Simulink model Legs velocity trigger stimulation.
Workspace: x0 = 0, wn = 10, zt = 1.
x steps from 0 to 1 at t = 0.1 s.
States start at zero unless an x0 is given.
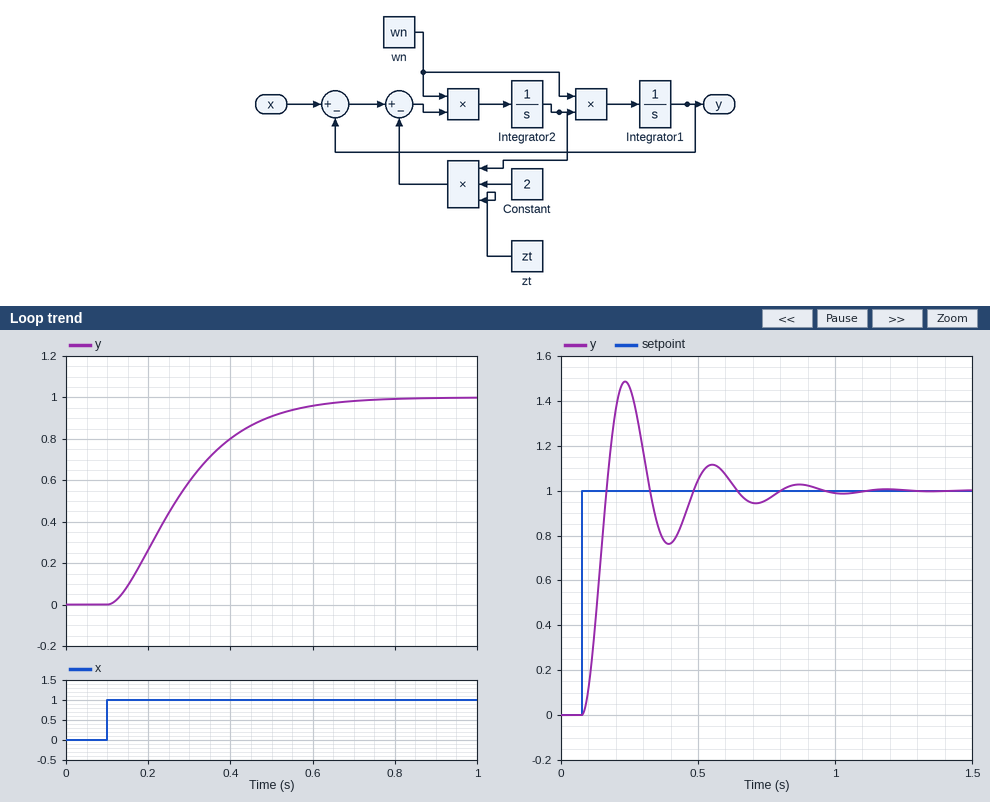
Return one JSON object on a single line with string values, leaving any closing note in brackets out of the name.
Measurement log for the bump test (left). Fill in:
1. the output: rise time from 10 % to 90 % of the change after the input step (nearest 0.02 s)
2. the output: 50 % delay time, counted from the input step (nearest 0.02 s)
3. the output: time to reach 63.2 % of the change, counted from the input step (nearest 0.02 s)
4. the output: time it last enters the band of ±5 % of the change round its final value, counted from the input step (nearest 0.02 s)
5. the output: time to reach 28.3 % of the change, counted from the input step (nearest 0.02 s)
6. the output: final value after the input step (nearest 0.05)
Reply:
{"the output: rise time from 10 % to 90 % of the change after the input step": "0.34 s", "the output: 50 % delay time, counted from the input step": "0.16 s", "the output: time to reach 63.2 % of the change, counted from the input step": "0.22 s", "the output: time it last enters the band of ±5 % of the change round its final value, counted from the input step": "0.48 s", "the output: time to reach 28.3 % of the change, counted from the input step": "0.10 s", "the output: final value after the input step": "1.00"}
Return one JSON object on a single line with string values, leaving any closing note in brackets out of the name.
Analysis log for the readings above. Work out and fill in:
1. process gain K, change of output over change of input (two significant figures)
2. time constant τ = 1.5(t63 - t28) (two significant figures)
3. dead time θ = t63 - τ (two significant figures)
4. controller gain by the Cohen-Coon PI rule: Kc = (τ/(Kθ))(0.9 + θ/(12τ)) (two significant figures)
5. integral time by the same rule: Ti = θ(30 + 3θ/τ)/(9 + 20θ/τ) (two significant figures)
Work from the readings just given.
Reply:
{"process gain K, change of output over change of input": "1.0", "time constant τ = 1.5(t63 - t28)": "0.18 s", "dead time θ = t63 - τ": "0.040 s", "controller gain by the Cohen-Coon PI rule: Kc = (τ/(Kθ))(0.9 + θ/(12τ))": "4.1", "integral time by the same rule: Ti = θ(30 + 3θ/τ)/(9 + 20θ/τ)": "0.091 s"}
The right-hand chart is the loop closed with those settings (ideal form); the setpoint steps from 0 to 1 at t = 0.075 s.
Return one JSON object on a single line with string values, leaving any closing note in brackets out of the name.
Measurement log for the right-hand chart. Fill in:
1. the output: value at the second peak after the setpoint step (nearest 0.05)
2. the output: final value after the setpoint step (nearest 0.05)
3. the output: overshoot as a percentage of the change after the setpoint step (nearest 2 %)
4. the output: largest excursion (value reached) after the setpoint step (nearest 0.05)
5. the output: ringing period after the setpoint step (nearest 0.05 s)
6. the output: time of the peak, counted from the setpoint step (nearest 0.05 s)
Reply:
{"the output: value at the second peak after the setpoint step": "1.10", "the output: final value after the setpoint step": "1.00", "the output: overshoot as a percentage of the change after the setpoint step": "48 %", "the output: largest excursion (value reached) after the setpoint step": "1.50", "the output: ringing period after the setpoint step": "0.30 s", "the output: time of the peak, counted from the setpoint step": "0.15 s"}
